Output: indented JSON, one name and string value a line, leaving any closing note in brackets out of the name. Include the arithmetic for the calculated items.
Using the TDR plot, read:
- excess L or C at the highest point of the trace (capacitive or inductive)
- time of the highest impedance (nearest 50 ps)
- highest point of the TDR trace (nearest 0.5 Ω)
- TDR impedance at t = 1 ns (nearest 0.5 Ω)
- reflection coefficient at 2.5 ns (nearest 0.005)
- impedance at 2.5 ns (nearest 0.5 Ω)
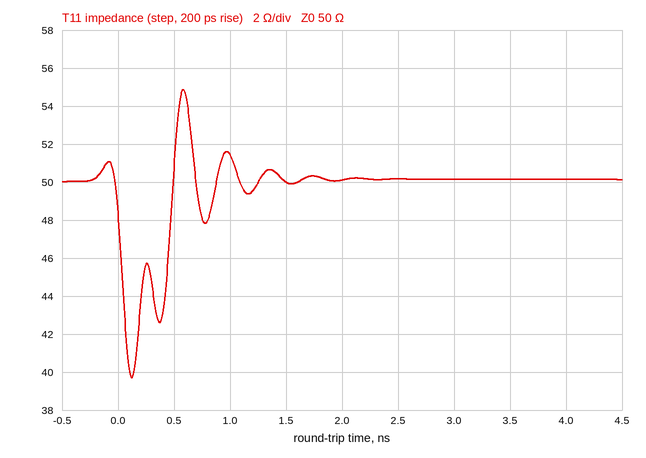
{
  "excess L or C at the highest point of the trace": "inductive",
  "time of the highest impedance": "600 ps",
  "highest point of the TDR trace": "55.0 Ω",
  "TDR impedance at t = 1 ns": "51.5 Ω",
  "reflection coefficient at 2.5 ns": "(50 − 50)/(50 + 50) ≈ 0.000",
  "impedance at 2.5 ns": "50.0 Ω"
}
